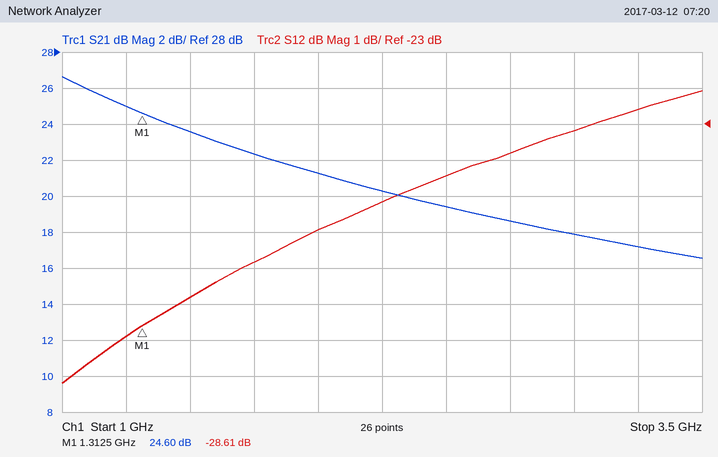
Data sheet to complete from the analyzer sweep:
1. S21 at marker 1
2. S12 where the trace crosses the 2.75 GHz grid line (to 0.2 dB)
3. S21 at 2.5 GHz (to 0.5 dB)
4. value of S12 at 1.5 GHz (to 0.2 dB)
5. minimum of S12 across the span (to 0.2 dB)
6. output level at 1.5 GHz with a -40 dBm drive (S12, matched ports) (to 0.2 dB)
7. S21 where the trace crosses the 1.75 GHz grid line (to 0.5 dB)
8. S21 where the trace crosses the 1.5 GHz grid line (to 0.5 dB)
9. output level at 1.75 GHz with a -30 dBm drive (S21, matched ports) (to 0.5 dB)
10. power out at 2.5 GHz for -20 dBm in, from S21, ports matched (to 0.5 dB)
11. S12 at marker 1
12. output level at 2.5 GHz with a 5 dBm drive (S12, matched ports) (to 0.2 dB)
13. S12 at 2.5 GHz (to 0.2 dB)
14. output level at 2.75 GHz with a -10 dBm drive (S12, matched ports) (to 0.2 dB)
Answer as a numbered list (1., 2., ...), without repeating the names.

1. 24.60 dB
2. -23.8 dB
3. 19.5 dB
4. -27.8 dB
5. -30.2 dB
6. -67.8 dBm
7. 22.5 dB
8. 23.5 dB
9. -7.5 dBm
10. -0.5 dBm
11. -28.61 dB
12. -19.4 dBm
13. -24.4 dB
14. -33.8 dBm
